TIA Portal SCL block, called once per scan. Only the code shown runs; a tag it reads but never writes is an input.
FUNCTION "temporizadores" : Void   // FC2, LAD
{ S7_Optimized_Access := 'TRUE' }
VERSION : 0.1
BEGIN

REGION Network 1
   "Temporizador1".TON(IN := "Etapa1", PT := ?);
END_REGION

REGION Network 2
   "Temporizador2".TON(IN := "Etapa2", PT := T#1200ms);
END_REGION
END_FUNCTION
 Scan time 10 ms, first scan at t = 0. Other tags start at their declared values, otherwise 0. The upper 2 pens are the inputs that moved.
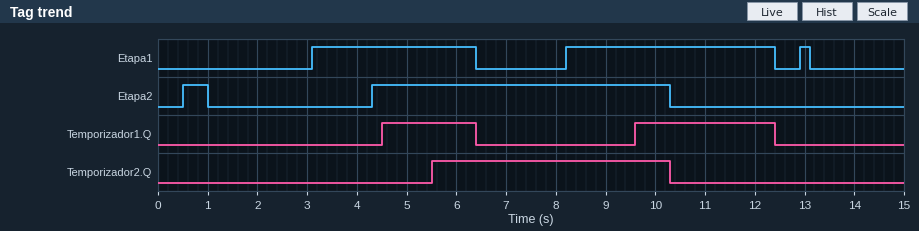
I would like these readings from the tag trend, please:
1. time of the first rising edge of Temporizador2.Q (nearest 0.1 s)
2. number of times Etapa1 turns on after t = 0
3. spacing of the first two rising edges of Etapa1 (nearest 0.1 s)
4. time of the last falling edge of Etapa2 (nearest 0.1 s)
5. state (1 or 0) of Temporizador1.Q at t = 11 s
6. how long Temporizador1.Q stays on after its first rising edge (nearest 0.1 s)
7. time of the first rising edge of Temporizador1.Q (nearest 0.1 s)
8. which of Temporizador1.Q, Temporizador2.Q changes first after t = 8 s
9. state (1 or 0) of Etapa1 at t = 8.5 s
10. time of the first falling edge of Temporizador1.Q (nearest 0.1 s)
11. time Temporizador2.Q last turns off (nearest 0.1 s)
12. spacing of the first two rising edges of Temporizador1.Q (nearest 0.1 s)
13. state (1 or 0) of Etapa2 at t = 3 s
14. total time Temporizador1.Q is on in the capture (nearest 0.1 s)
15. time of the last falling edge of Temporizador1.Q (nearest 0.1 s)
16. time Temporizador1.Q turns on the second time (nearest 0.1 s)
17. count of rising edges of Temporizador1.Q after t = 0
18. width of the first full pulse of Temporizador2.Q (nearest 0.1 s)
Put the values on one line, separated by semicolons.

5.5 s; 3; 5.1 s; 10.3 s; 1; 1.9 s; 4.5 s; Temporizador1.Q; 1; 6.4 s; 10.3 s; 5.1 s; 0; 4.7 s; 12.4 s; 9.6 s; 2; 4.8 s
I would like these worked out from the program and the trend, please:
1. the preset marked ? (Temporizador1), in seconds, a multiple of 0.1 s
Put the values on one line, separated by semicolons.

1.4 s
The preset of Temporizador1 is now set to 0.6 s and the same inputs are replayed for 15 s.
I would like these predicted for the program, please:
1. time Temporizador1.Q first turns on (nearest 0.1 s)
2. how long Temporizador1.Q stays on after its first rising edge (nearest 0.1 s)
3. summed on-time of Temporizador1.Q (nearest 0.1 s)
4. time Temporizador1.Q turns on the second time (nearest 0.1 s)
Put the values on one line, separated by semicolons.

3.7 s; 2.7 s; 6.3 s; 8.8 s
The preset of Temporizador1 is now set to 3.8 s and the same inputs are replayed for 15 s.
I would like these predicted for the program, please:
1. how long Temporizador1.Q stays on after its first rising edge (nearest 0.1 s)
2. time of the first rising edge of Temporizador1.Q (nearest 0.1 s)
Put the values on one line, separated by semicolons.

0.4 s; 12.0 s
